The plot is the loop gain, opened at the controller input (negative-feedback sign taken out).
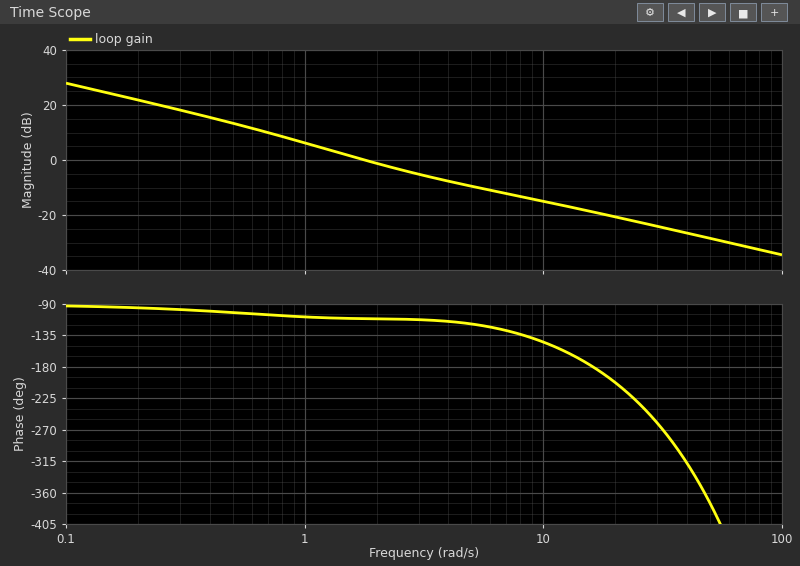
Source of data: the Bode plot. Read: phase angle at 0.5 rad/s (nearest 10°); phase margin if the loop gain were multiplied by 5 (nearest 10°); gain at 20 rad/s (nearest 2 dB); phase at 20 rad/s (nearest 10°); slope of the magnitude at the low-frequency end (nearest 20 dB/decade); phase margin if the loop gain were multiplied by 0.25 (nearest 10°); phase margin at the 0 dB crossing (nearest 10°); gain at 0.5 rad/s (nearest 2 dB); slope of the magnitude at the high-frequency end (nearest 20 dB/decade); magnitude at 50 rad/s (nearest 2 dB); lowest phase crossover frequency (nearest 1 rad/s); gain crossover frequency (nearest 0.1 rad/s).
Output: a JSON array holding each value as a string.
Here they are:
["-100°", "40°", "-20 dB", "-200°", "-20 dB/decade", "80°", "70°", "14 dB", "-20 dB/decade", "-28 dB", "16 rad/s", "1.8 rad/s"]
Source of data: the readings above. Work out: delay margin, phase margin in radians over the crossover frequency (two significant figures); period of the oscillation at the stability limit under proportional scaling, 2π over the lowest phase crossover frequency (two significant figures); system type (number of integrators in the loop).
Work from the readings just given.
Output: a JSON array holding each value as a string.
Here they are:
["0.68 s", "0.39 s", "1"]
